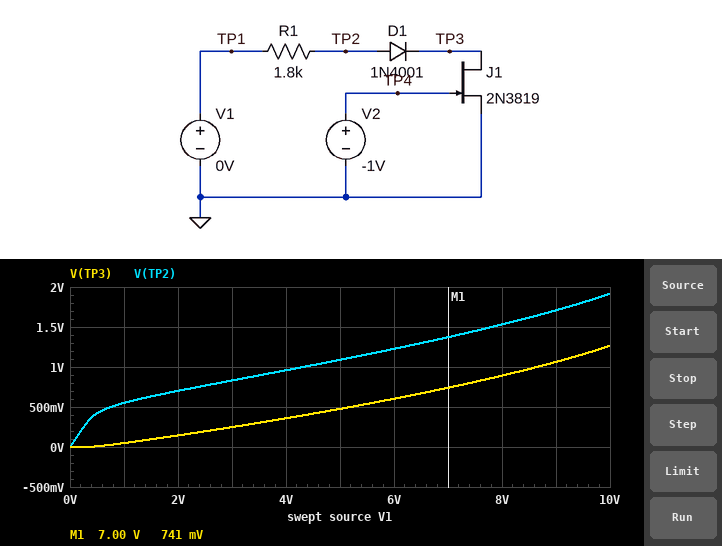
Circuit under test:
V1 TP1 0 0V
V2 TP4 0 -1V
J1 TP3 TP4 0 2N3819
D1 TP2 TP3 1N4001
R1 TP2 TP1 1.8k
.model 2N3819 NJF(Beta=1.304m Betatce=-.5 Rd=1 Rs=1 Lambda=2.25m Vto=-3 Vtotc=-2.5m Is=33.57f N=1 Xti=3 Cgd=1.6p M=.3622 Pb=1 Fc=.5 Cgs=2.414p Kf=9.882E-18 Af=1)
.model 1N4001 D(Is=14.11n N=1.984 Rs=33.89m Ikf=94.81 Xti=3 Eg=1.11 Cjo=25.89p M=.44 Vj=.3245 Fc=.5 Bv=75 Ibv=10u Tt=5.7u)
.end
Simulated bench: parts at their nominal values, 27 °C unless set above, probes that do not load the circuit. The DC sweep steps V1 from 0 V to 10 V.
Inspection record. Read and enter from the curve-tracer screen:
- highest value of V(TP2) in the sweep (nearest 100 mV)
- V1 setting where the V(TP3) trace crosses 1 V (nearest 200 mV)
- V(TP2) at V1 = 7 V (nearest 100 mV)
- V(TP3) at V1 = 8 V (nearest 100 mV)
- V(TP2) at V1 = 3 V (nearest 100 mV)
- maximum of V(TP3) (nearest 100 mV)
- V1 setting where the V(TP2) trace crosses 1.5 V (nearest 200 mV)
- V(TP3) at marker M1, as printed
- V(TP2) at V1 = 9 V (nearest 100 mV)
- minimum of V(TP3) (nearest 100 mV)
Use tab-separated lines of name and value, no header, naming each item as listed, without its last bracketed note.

highest value of V(TP2) in the sweep	1.9 V
V1 setting where the V(TP3) trace crosses 1 V	8.6 V
V(TP2) at V1 = 7 V	1.4 V
V(TP3) at V1 = 8 V	900 mV
V(TP2) at V1 = 3 V	800 mV
maximum of V(TP3)	1.3 V
V1 setting where the V(TP2) trace crosses 1.5 V	7.8 V
V(TP3) at marker M1, as printed	741 mV
V(TP2) at V1 = 9 V	1.7 V
minimum of V(TP3)	0 V
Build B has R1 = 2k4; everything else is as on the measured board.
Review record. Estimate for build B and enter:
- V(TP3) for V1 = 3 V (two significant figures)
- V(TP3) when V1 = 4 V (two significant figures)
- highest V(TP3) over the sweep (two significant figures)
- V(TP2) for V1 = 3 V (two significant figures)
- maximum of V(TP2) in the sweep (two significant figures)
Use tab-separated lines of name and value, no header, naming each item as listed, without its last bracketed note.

V(TP3) for V1 = 3 V	190 mV
V(TP3) when V1 = 4 V	270 mV
highest V(TP3) over the sweep	870 mV
V(TP2) for V1 = 3 V	760 mV
maximum of V(TP2) in the sweep	1.5 V
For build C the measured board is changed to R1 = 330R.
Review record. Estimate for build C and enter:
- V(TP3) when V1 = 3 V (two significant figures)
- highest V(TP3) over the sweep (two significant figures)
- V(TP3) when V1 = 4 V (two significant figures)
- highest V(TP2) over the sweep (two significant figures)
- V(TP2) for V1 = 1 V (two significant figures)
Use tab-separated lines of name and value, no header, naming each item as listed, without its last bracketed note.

V(TP3) when V1 = 3 V	1.0 V
highest V(TP3) over the sweep	7.6 V
V(TP3) when V1 = 4 V	1.7 V
highest V(TP2) over the sweep	8.3 V
V(TP2) for V1 = 1 V	730 mV
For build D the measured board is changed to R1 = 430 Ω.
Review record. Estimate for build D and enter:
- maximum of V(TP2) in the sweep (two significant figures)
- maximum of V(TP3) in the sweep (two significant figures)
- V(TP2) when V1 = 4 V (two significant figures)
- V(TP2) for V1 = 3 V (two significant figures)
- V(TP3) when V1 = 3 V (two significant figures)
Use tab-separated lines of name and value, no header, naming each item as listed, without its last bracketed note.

maximum of V(TP2) in the sweep	7.7 V
maximum of V(TP3) in the sweep	7.1 V
V(TP2) when V1 = 4 V	2.0 V
V(TP2) for V1 = 3 V	1.5 V
V(TP3) when V1 = 3 V	860 mV
